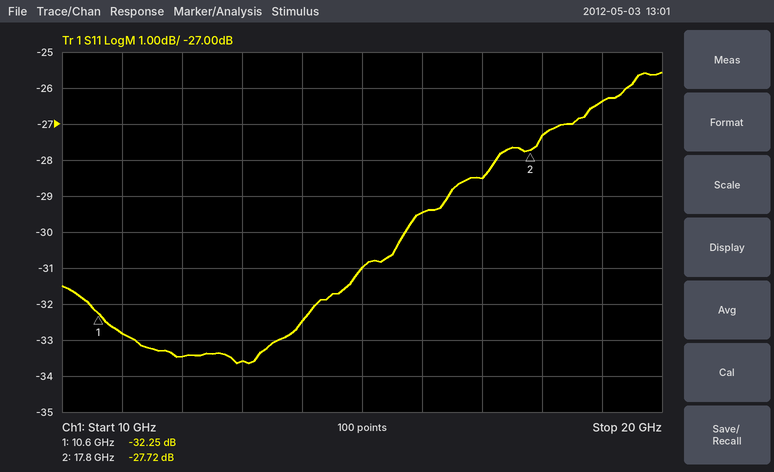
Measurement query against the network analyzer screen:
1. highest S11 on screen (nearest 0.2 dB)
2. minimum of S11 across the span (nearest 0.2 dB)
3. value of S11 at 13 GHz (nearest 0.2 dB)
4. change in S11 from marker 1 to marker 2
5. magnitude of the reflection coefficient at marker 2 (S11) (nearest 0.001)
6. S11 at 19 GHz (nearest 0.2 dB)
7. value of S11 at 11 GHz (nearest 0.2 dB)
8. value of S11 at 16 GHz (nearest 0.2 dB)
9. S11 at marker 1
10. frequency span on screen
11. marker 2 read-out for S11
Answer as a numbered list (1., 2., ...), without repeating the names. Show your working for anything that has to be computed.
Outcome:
1. -25.6 dB
2. -33.6 dB
3. -33.6 dB
4. -27.72 − (-32.25) = 4.53 dB
5. 10^(-27.72/20) ≈ 0.041
6. -26.4 dB
7. -32.8 dB
8. -29.4 dB
9. -32.25 dB
10. 10 GHz
11. -27.72 dB
